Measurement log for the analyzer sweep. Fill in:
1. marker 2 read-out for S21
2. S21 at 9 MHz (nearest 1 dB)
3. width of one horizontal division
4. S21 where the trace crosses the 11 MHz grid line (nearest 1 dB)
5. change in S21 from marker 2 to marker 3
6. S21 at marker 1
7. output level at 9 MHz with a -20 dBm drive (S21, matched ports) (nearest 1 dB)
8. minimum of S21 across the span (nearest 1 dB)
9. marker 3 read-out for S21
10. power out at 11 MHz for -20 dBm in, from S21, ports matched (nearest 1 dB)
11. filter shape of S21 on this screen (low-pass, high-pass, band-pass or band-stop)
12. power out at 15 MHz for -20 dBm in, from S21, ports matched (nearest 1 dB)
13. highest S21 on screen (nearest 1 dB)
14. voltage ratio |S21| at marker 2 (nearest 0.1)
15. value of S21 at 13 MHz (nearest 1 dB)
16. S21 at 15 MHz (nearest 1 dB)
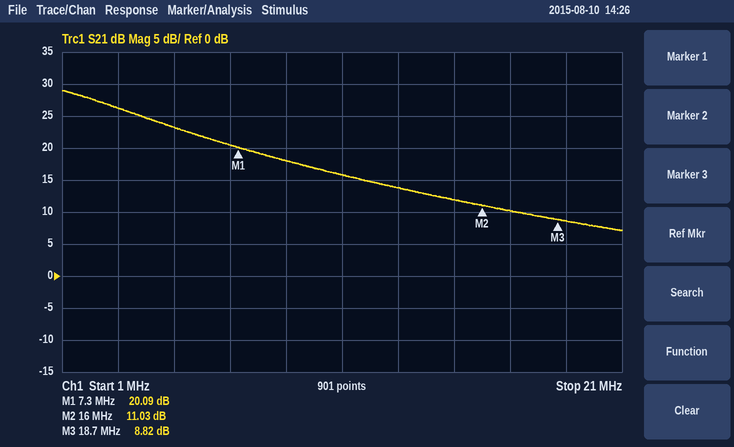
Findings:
11.03 dB
18 dB
2 MHz
16 dB
-2.21 dB
20.09 dB
-2 dBm
7 dB
8.82 dB
-4 dBm
low-pass
-8 dBm
29 dB
3.6
14 dB
12 dB
